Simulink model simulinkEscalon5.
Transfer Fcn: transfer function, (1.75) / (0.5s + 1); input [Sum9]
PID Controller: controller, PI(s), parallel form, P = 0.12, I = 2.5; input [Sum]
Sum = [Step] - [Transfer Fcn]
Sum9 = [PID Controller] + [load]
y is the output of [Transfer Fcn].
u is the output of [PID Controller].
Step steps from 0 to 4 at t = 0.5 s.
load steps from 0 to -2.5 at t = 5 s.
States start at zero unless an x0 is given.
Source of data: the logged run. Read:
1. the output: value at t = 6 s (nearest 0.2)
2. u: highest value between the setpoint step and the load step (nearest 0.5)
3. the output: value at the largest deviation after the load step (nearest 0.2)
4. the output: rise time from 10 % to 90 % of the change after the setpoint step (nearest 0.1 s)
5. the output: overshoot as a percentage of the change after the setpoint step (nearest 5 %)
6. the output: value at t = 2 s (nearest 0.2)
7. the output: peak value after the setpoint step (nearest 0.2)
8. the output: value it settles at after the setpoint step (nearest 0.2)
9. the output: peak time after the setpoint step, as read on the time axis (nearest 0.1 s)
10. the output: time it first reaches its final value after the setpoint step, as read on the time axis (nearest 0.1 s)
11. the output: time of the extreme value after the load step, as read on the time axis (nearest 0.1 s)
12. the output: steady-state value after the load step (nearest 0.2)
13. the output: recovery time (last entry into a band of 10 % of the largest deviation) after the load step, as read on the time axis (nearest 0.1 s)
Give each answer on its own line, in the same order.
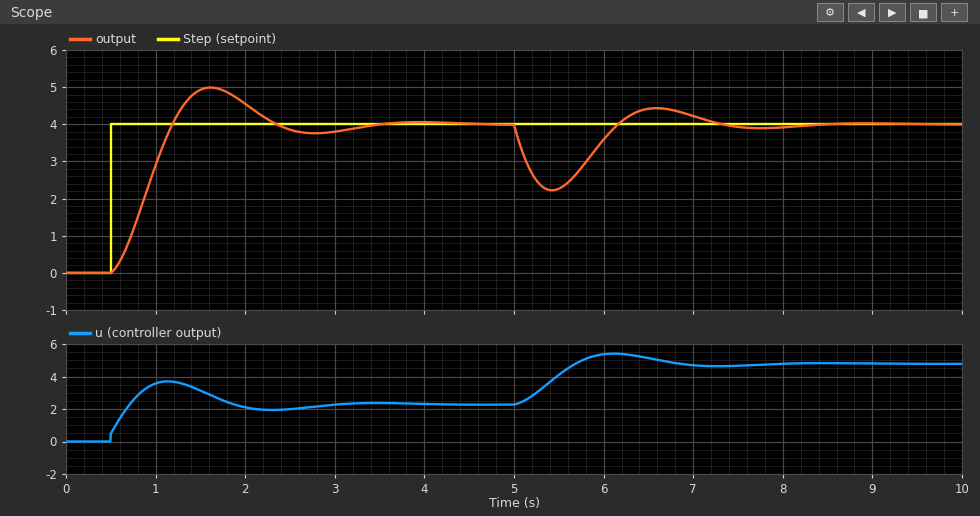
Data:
3.6
3.5
2.2
0.5 s
25 %
4.6
5.0
4.0
1.6 s
1.2 s
5.4 s
4.0
7.1 s
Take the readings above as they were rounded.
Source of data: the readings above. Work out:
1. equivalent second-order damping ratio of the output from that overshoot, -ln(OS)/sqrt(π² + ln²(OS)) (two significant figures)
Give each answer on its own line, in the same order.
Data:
0.40
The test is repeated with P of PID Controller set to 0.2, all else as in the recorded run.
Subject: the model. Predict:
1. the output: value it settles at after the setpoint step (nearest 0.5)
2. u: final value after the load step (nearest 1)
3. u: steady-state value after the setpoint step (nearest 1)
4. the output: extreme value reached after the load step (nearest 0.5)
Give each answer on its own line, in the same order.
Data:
4.0
5
2
2.5
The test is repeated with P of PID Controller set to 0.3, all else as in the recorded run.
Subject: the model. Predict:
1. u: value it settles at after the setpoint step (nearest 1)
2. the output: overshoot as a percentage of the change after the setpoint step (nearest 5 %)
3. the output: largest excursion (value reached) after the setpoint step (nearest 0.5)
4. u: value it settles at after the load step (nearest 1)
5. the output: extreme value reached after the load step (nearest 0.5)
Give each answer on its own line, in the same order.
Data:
2
15 %
4.5
5
2.5
